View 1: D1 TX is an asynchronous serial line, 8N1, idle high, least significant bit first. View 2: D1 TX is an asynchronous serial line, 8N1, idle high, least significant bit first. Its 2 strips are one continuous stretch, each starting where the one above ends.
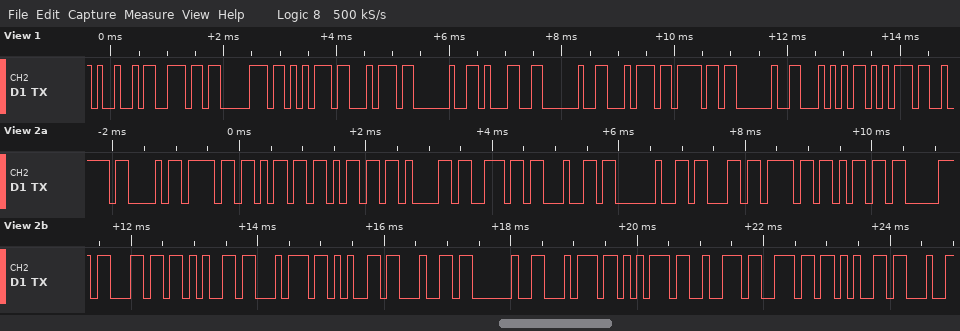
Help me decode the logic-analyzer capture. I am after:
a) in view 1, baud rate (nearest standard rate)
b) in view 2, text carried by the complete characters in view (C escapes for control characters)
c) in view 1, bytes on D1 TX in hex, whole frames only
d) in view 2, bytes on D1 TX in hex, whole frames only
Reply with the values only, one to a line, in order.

9600 baud
"Command completed turne"
49 6E 70 75 74 20 31 20 74 6F 20 54 75
43 6F 6D 6D 61 6E 64 20 63 6F 6D 70 6C 65 74 65 64 20 74 75 72 6E 65
